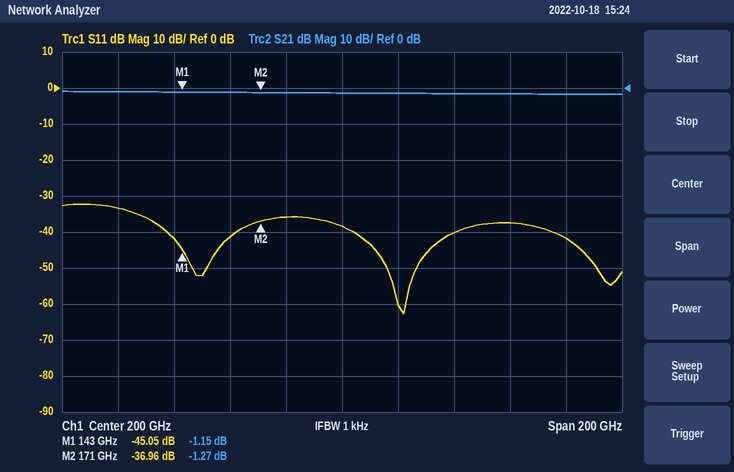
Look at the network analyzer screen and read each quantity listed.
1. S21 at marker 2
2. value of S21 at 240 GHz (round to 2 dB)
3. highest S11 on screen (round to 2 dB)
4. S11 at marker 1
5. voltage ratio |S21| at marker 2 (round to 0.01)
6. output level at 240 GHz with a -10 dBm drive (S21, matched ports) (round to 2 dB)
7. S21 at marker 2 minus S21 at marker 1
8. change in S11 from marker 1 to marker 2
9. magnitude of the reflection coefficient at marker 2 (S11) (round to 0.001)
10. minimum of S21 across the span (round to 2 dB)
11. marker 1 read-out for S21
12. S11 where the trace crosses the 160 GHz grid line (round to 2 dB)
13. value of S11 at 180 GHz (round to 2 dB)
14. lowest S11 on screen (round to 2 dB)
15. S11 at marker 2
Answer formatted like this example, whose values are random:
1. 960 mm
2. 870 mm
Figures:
1. -1.27 dB
2. -2 dB
3. -32 dB
4. -45.05 dB
5. 0.86
6. -12 dBm
7. -0.12 dB
8. 8.09 dB
9. 0.014
10. -2 dB
11. -1.15 dB
12. -42 dB
13. -36 dB
14. -62 dB
15. -36.96 dB
